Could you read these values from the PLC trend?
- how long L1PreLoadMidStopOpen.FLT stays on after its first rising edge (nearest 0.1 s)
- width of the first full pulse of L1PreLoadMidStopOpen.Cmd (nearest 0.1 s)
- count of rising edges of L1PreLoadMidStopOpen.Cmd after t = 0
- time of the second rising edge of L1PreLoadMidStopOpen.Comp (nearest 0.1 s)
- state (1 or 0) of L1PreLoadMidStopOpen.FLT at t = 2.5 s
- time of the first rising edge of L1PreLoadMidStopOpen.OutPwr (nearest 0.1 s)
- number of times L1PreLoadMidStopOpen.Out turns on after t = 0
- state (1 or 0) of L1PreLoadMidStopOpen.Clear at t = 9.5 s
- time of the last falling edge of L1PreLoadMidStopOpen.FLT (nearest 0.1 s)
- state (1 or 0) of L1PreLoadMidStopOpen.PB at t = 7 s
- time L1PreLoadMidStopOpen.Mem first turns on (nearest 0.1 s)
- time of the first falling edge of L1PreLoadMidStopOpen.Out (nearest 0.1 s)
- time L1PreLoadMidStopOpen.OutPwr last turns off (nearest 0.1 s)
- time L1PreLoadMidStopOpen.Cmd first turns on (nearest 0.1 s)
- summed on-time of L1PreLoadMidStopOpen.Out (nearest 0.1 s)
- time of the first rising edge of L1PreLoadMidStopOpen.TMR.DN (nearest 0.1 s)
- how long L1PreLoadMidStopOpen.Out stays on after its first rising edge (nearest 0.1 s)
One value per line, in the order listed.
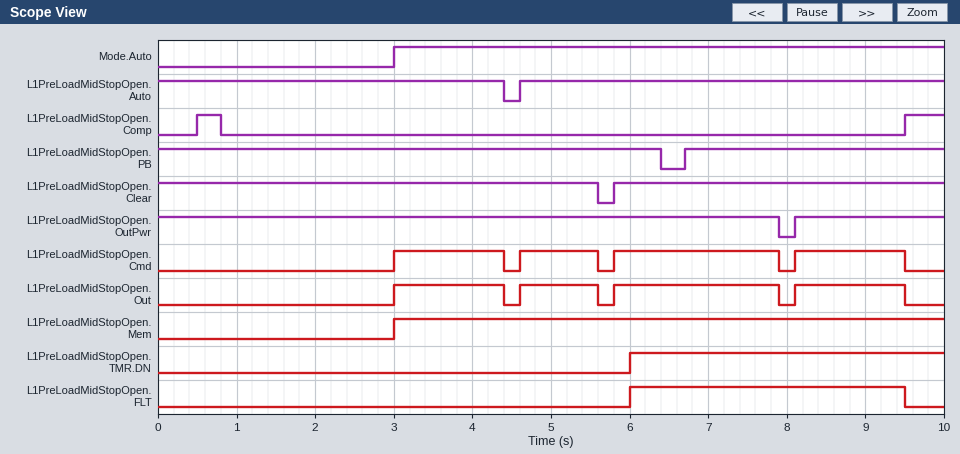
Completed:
3.5 s
1.4 s
4
9.5 s
0
8.1 s
4
1
9.5 s
1
3.0 s
4.4 s
7.9 s
3.0 s
5.9 s
6.0 s
1.4 s
